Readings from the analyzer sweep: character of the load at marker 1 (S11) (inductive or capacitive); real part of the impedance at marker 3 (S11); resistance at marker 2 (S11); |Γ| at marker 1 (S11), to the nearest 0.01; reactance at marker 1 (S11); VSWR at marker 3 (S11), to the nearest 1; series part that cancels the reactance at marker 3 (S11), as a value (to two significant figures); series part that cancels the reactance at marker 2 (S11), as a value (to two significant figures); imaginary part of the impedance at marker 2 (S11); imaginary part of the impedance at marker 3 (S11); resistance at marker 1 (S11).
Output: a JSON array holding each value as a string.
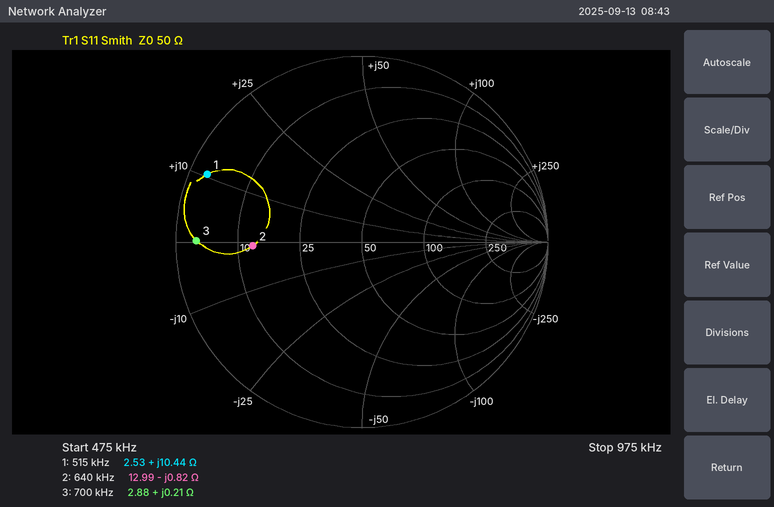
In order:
["inductive", "2.88 Ω", "12.99 Ω", "0.91", "+10.44 Ω", "17", "1.1 µF", "200 nH", "-0.82 Ω", "+0.21 Ω", "2.53 Ω"]
